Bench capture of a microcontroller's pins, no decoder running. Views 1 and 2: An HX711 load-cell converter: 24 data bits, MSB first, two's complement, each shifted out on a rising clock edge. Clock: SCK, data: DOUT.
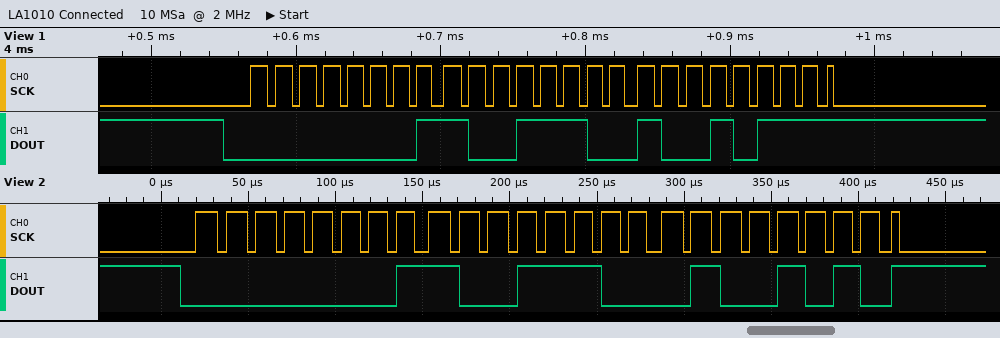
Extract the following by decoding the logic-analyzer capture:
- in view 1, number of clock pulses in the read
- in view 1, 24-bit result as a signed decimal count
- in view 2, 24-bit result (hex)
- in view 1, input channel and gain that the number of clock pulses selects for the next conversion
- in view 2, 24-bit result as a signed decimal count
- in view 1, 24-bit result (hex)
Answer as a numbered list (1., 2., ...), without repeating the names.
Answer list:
1. 25
2. 105623
3. 0x019C4A
4. channel A, gain 128
5. 105546
6. 0x019C97
